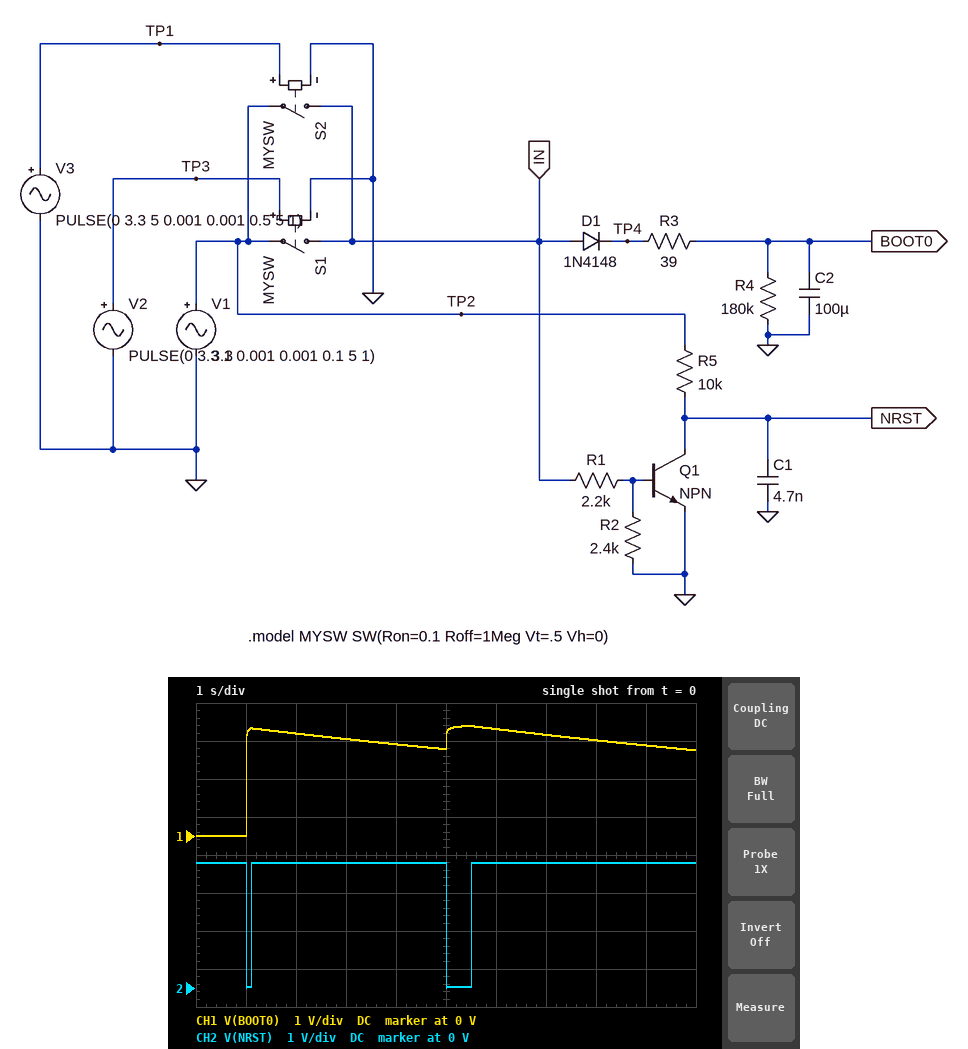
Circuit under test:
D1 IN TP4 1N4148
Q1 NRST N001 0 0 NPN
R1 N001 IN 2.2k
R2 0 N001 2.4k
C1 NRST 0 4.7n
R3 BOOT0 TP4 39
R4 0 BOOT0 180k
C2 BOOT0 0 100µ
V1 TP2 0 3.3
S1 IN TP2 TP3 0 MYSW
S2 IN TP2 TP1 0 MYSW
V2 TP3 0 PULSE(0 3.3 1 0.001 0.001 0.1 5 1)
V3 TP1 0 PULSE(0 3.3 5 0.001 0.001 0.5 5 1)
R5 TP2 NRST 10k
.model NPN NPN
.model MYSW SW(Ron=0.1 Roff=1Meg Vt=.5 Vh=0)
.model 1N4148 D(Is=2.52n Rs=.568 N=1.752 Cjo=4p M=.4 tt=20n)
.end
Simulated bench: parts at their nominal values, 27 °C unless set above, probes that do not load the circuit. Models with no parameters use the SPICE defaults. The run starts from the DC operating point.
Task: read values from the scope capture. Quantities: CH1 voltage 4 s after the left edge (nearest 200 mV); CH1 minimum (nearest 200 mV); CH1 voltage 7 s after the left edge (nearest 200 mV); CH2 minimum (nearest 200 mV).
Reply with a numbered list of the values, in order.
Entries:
1. 2.4 V
2. 0 V
3. 2.6 V
4. 0 V
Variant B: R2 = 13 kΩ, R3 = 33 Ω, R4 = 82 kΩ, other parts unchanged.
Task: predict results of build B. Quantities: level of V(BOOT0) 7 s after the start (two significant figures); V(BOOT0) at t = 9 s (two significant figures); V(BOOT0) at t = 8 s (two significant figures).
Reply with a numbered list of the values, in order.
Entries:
1. 2.4 V
2. 1.9 V
3. 2.1 V
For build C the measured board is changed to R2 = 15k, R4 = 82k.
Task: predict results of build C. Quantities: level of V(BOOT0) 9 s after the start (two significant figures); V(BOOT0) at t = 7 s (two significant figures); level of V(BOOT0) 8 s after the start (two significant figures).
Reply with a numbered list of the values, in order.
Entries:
1. 1.9 V
2. 2.4 V
3. 2.1 V
